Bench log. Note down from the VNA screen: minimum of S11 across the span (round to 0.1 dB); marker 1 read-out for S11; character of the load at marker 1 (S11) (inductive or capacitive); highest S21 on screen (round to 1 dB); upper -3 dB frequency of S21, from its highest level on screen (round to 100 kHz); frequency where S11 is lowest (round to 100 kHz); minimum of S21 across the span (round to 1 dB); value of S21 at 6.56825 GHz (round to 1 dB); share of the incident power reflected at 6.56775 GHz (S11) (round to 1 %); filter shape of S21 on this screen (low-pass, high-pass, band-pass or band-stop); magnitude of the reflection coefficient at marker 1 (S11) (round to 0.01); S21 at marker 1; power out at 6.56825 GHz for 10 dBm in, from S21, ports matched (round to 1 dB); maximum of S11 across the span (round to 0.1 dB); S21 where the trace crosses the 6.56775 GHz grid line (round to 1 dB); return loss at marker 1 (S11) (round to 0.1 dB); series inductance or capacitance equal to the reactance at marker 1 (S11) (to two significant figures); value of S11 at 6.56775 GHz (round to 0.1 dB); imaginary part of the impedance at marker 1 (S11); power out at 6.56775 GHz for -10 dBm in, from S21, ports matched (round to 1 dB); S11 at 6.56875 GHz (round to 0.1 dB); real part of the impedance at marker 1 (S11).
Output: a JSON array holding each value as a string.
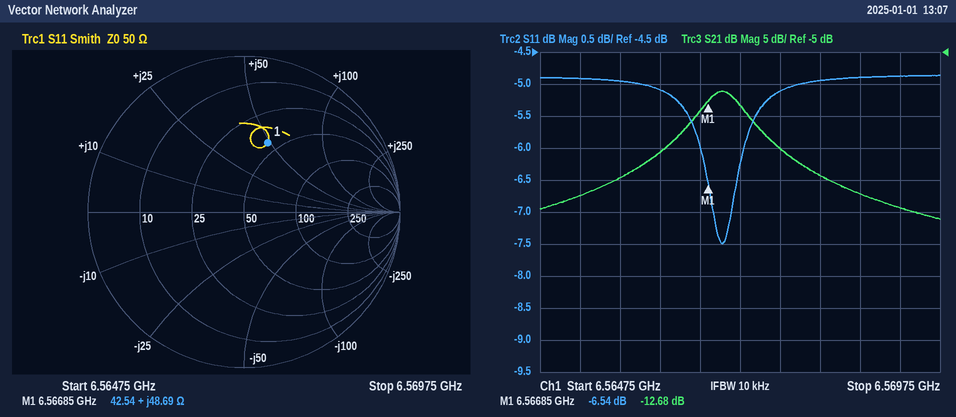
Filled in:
["-7.5 dB", "-6.54 dB", "inductive", "-11 dB", "6.5673 GHz", "6.5670 GHz", "-31 dB", "-24 dB", "31 %", "band-pass", "0.47", "-12.68 dB", "-14 dBm", "-4.9 dB", "-20 dB", "6.5 dB", "1.2 nH", "-5.1 dB", "+48.69 Ω", "-30 dBm", "-4.9 dB", "42.54 Ω"]
